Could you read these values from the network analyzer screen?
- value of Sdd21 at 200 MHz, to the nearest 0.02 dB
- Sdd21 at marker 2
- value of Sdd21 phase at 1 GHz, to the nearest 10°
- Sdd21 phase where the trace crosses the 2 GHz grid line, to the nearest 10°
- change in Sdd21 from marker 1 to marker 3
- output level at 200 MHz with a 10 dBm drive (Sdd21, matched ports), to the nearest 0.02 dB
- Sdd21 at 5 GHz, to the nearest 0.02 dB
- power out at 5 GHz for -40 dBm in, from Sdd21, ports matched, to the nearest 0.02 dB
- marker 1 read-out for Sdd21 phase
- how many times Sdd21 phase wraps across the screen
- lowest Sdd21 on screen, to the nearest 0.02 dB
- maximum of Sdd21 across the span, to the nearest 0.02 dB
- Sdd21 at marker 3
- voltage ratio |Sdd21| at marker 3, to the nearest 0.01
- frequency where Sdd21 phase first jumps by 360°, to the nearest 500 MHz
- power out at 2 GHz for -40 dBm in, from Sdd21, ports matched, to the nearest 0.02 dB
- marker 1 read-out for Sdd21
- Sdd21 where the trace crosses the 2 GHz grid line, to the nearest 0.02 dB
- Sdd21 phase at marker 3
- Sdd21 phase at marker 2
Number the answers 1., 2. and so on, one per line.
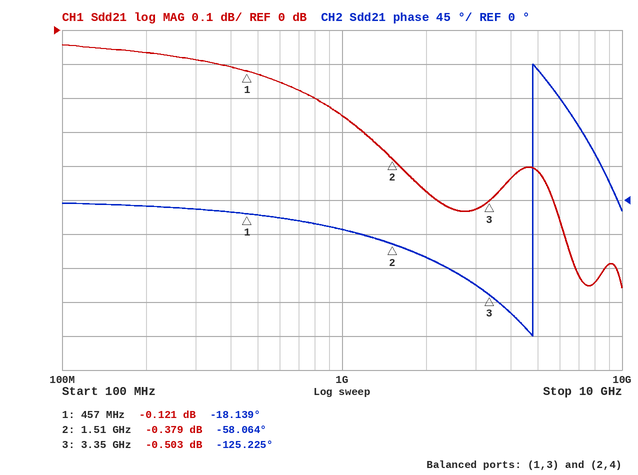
1. -0.06 dB
2. -0.379 dB
3. -40°
4. -80°
5. -0.382 dB
6. 9.94 dBm
7. -0.42 dB
8. -40.42 dBm
9. -18.139°
10. 1
11. -0.76 dB
12. -0.04 dB
13. -0.503 dB
14. 0.94
15. 5.0 GHz
16. -40.48 dBm
17. -0.121 dB
18. -0.48 dB
19. -125.225°
20. -58.064°
